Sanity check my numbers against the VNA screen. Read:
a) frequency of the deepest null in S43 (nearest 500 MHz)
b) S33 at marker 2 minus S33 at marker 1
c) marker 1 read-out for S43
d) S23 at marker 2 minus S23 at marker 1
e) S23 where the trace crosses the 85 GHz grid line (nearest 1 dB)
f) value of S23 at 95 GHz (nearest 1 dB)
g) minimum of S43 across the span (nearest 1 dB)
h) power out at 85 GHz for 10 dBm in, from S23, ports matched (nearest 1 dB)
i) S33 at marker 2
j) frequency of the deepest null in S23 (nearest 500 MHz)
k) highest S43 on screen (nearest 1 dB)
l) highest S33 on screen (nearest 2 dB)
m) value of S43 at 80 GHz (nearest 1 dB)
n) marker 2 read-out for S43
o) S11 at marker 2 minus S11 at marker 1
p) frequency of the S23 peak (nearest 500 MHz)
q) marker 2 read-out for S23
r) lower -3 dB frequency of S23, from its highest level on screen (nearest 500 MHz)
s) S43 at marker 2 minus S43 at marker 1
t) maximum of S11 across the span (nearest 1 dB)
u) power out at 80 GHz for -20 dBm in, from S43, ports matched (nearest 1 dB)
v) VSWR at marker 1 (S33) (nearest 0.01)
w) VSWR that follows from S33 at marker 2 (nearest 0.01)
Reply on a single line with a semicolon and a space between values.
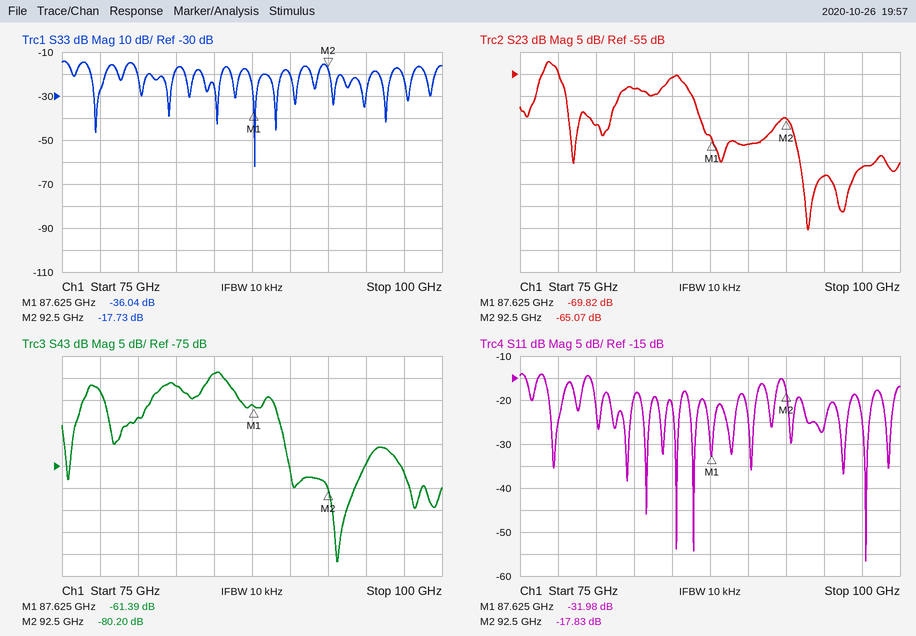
93.0 GHz; 18.31 dB; -61.39 dB; 4.75 dB; -56 dB; -78 dB; -97 dB; -46 dBm; -17.73 dB; 94.0 GHz; -54 dB; -14 dB; -64 dB; -80.20 dB; 14.15 dB; 77.0 GHz; -65.07 dB; 76.5 GHz; -18.81 dB; -14 dB; -84 dBm; 1.03; 1.30
